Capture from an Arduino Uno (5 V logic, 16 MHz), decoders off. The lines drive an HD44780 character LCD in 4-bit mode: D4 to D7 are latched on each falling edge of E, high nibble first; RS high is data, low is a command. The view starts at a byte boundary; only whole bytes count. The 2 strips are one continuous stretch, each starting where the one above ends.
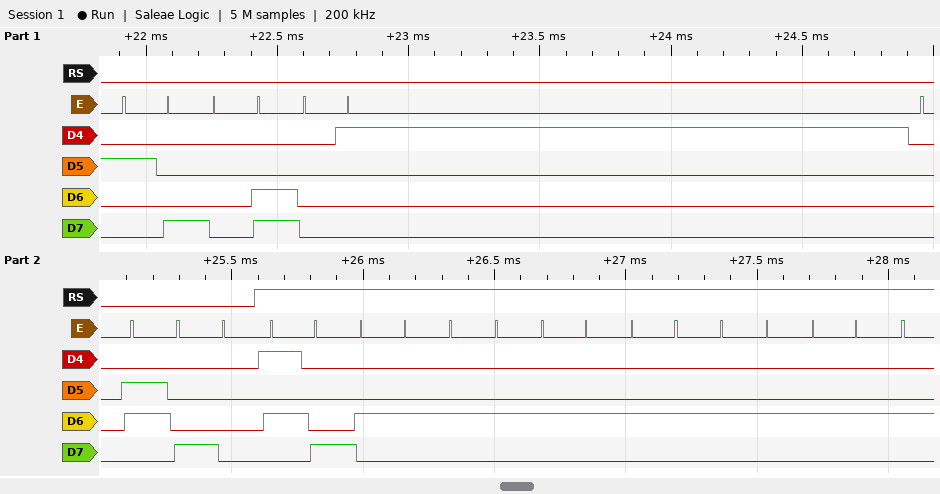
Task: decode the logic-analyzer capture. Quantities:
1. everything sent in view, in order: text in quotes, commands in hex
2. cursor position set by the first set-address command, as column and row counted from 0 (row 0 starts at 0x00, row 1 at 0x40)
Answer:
0x28 0x0C 0x01 0x06 0x80 "XDDDDDD"
column 0, row 0
